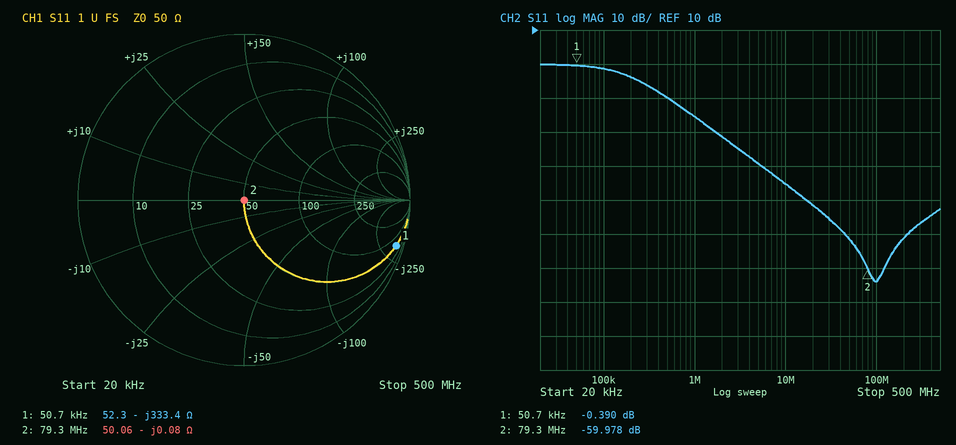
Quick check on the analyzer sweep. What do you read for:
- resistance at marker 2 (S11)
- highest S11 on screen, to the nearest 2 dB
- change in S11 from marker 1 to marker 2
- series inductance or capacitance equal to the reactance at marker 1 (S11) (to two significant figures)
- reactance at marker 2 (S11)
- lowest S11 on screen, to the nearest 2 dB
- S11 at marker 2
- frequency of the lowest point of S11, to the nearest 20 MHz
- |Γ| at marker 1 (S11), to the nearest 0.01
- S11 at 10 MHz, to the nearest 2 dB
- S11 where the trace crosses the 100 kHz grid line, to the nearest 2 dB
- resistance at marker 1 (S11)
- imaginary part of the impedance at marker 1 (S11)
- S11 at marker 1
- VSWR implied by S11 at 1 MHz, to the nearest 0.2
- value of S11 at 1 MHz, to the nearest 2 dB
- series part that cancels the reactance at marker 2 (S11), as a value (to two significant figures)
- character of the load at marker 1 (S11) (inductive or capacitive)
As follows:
50.06 Ω
0 dB
-59.588 dB
9.4 nF
-0.08 Ω
-64 dB
-59.978 dB
100 MHz
0.96
-36 dB
-2 dB
52.3 Ω
-333.4 Ω
-0.390 dB
1.4
-16 dB
160 pH
capacitive
